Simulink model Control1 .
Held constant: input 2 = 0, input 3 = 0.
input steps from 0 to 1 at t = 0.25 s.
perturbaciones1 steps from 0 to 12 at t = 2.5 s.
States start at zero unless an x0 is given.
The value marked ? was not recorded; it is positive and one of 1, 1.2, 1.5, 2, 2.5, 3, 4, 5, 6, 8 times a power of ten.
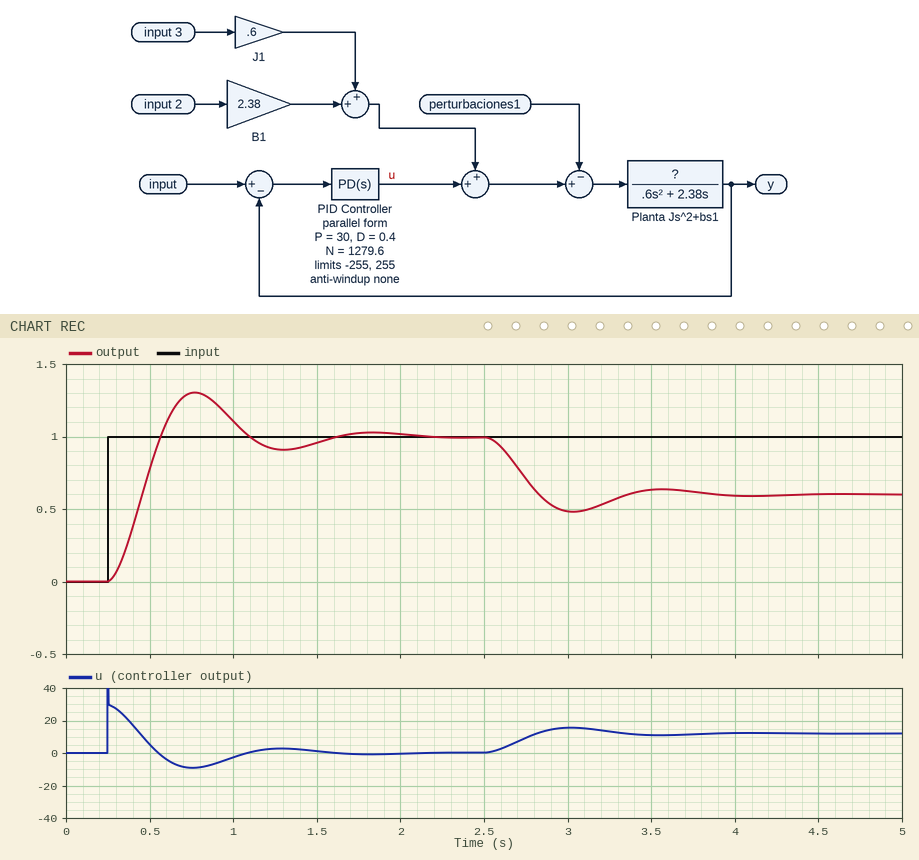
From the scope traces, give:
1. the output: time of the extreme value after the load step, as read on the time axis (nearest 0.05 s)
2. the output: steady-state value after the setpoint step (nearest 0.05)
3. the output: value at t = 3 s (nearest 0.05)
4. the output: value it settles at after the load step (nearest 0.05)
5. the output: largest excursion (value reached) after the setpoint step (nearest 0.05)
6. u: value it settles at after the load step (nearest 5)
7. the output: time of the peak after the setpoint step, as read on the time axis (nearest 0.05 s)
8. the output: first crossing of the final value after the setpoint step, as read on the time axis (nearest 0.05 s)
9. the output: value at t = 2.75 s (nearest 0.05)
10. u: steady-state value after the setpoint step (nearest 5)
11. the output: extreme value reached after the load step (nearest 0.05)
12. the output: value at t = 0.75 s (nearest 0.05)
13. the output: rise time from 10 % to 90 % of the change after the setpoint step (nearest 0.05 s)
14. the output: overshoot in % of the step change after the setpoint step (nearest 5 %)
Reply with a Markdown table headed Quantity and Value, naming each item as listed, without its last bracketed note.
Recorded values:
| Quantity | Value |
|---|---|
| the output: time of the extreme value after the load step, as read on the time axis | 3.05 s |
| the output: steady-state value after the setpoint step | 1.00 |
| the output: value at t = 3 s | 0.50 |
| the output: value it settles at after the load step | 0.60 |
| the output: largest excursion (value reached) after the setpoint step | 1.30 |
| u: value it settles at after the load step | 10 |
| the output: time of the peak after the setpoint step, as read on the time axis | 0.75 s |
| the output: first crossing of the final value after the setpoint step, as read on the time axis | 0.55 s |
| the output: value at t = 2.75 s | 0.70 |
| u: steady-state value after the setpoint step | 0 |
| the output: extreme value reached after the load step | 0.50 |
| the output: value at t = 0.75 s | 1.30 |
| the output: rise time from 10 % to 90 % of the change after the setpoint step | 0.20 s |
| the output: overshoot in % of the step change after the setpoint step | 30 % |
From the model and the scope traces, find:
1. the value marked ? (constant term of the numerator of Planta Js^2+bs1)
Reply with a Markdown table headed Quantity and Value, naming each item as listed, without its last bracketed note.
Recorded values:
| Quantity | Value |
|---|---|
| the value marked ? | 0.8 |
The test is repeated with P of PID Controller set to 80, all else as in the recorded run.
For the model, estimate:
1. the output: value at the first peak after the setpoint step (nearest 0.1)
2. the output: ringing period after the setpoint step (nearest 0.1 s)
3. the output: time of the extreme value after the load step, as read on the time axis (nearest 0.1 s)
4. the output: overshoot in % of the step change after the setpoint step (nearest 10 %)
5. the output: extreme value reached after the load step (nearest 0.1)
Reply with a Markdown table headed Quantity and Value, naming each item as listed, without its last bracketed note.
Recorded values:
| Quantity | Value |
|---|---|
| the output: value at the first peak after the setpoint step | 1.5 |
| the output: ringing period after the setpoint step | 0.6 s |
| the output: time of the extreme value after the load step, as read on the time axis | 2.8 s |
| the output: overshoot in % of the step change after the setpoint step | 50 % |
| the output: extreme value reached after the load step | 0.8 |
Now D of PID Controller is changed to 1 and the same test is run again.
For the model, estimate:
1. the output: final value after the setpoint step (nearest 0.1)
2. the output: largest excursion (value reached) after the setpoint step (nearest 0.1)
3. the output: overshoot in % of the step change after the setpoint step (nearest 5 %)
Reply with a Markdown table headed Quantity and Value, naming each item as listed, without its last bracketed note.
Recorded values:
| Quantity | Value |
|---|---|
| the output: final value after the setpoint step | 1.0 |
| the output: largest excursion (value reached) after the setpoint step | 1.2 |
| the output: overshoot in % of the step change after the setpoint step | 25 % |
